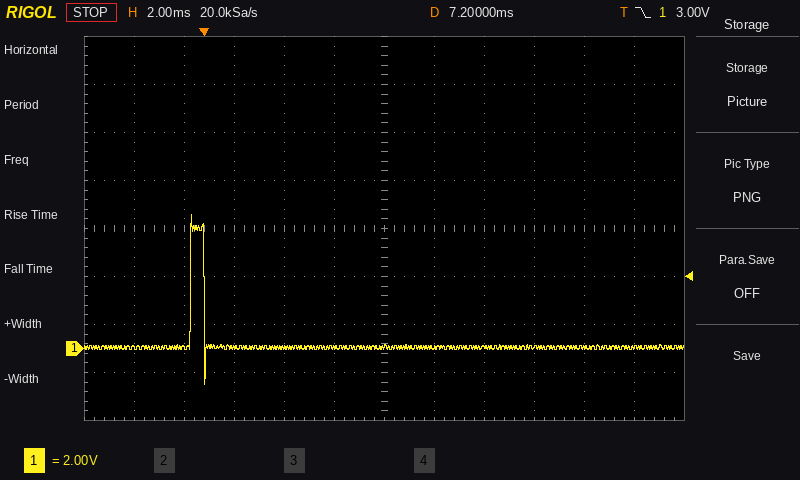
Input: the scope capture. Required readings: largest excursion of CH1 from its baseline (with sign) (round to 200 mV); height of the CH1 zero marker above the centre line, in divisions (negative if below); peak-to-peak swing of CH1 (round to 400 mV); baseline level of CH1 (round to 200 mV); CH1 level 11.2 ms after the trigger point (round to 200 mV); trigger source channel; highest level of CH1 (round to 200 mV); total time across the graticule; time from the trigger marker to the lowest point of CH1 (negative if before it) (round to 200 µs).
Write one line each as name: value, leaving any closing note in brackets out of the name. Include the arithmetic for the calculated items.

largest excursion of CH1 from its baseline (with sign): 5.6 V − (0.0 V) = +5.6 V
height of the CH1 zero marker above the centre line, in divisions: -2.5 div
peak-to-peak swing of CH1: 7.2 V
baseline level of CH1: 0.0 V
CH1 level 11.2 ms after the trigger point: 0.0 V
trigger source channel: CH1
highest level of CH1: 5.6 V
total time across the graticule: 24 ms
time from the trigger marker to the lowest point of CH1 (negative if before it): 0.0 ms
